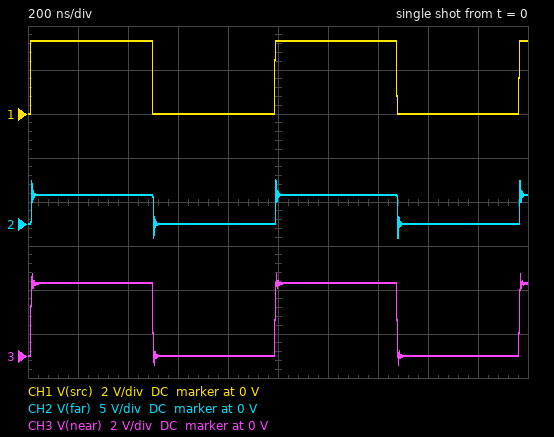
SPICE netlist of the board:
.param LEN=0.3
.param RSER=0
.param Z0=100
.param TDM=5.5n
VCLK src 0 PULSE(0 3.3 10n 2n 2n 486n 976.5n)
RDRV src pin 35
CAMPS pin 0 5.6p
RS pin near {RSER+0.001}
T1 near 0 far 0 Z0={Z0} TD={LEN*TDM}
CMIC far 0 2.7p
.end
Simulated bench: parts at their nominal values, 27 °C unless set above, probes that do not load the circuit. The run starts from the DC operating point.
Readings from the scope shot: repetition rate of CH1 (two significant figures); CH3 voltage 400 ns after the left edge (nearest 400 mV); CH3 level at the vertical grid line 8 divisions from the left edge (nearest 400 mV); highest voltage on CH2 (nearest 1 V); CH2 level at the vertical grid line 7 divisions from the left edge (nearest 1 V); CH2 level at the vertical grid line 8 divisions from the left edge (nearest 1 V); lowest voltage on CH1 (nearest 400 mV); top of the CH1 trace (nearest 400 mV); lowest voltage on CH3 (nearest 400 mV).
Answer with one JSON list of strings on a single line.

["1.0 MHz", "3.2 V", "0 V", "5 V", "3 V", "0 V", "0 V", "3.2 V", "-400 mV"]
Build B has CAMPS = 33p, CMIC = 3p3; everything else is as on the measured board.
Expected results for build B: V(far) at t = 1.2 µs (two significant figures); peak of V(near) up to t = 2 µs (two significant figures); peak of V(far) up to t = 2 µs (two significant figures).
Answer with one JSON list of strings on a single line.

["3.3 V", "3.6 V", "4.7 V"]
